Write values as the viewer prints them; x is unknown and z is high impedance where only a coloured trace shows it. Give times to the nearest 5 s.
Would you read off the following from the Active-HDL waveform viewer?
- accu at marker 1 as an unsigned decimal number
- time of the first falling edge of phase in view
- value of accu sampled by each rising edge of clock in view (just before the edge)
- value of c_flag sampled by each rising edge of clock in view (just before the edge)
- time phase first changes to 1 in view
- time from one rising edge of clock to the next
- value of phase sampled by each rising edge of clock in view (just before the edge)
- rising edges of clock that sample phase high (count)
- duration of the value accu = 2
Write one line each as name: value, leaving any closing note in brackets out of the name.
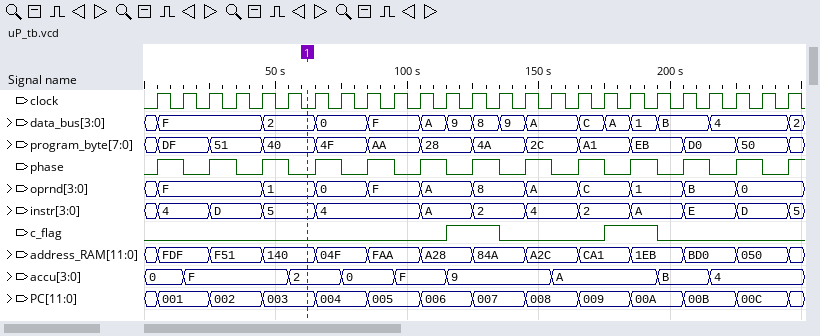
accu at marker 1 as an unsigned decimal number: 2
time of the first falling edge of phase in view: 15 s
value of accu sampled by each rising edge of clock in view: 0, 0, F, F, F, F, 2, 2, 0, 0, F, F, 9, 9, 9, 9, A, A, A, A, B, B, 4, 4, 4
value of c_flag sampled by each rising edge of clock in view: 0 0 0 0 0 0 0 0 0 0 0 0 1 1 0 0 0 0 1 1 0 0 0 0 0
time phase first changes to 1 in view: 5 s
time from one rising edge of clock to the next: 10 s
value of phase sampled by each rising edge of clock in view: 0 1 0 1 0 1 0 1 0 1 0 1 0 1 0 1 0 1 0 1 0 1 0 1 0
rising edges of clock that sample phase high: 12
duration of the value accu = 2: 20 s
